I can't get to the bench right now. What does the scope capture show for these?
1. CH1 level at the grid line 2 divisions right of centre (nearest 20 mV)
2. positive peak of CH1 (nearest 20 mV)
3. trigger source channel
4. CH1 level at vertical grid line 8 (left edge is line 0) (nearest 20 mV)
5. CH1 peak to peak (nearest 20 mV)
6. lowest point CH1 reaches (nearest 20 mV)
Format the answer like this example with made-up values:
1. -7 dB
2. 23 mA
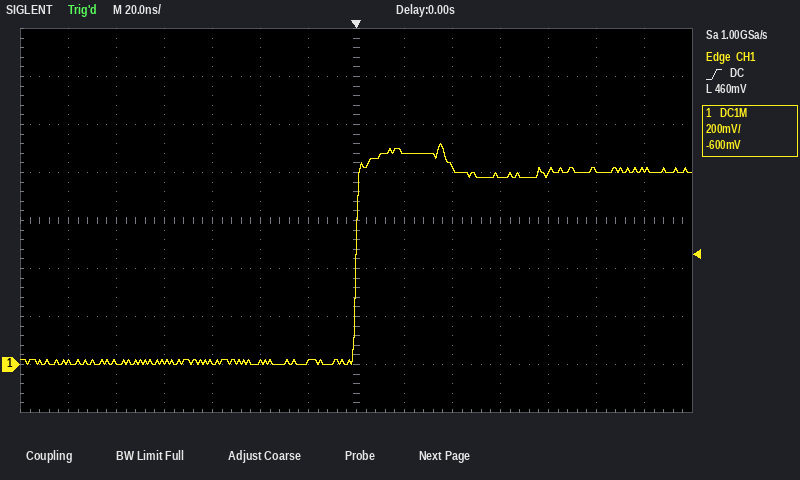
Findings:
1. 820 mV
2. 920 mV
3. CH1
4. 880 mV
5. 920 mV
6. 0 mV
